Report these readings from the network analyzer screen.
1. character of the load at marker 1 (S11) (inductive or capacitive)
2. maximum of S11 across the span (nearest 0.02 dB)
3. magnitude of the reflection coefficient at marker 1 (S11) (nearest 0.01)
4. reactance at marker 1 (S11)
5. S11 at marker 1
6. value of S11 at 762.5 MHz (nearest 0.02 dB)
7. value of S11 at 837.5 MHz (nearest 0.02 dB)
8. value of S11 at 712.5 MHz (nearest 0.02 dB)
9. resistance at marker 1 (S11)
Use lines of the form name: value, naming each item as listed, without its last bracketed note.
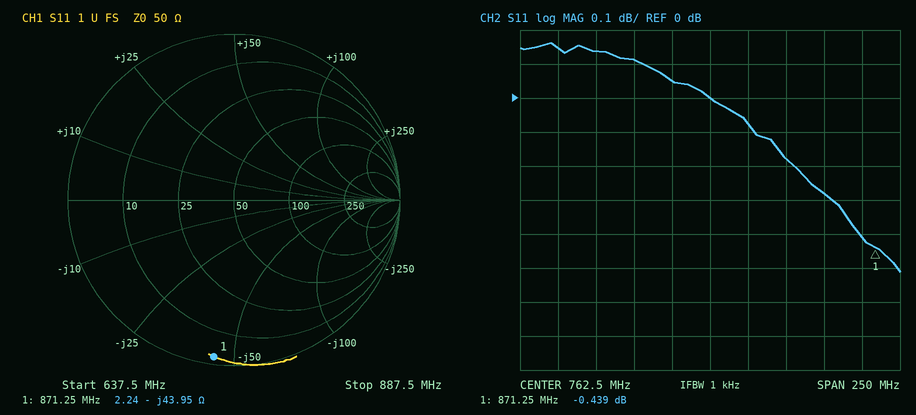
character of the load at marker 1 (S11): capacitive
maximum of S11 across the span: 0.16 dB
magnitude of the reflection coefficient at marker 1 (S11): 0.95
reactance at marker 1: -43.95 Ω
S11 at marker 1: -0.439 dB
value of S11 at 762.5 MHz: 0.00 dB
value of S11 at 837.5 MHz: -0.28 dB
value of S11 at 712.5 MHz: 0.12 dB
resistance at marker 1: 2.24 Ω
